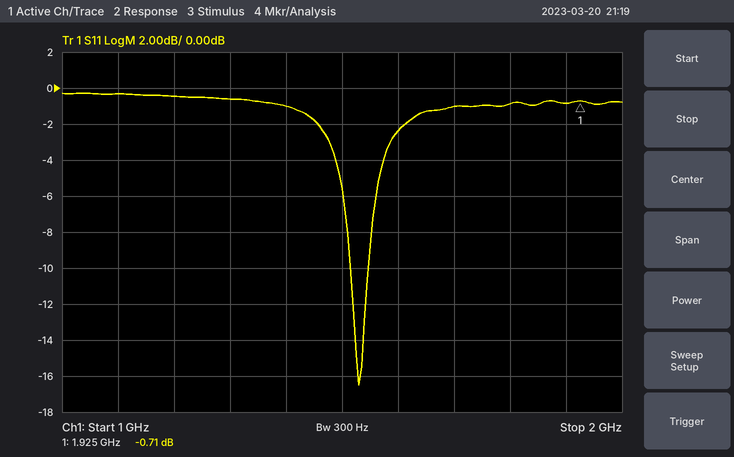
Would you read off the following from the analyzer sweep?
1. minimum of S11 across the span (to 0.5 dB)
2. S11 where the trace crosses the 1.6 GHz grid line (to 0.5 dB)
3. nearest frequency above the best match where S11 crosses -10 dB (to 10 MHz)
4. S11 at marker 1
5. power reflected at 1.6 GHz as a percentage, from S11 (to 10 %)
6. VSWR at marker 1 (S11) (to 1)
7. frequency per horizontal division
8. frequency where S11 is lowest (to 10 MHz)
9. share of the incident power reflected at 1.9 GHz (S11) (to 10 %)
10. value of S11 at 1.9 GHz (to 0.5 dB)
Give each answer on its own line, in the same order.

-16.5 dB
-2.5 dB
1.55 GHz
-0.71 dB
60 %
24
100 MHz
1.53 GHz
80 %
-1.0 dB
